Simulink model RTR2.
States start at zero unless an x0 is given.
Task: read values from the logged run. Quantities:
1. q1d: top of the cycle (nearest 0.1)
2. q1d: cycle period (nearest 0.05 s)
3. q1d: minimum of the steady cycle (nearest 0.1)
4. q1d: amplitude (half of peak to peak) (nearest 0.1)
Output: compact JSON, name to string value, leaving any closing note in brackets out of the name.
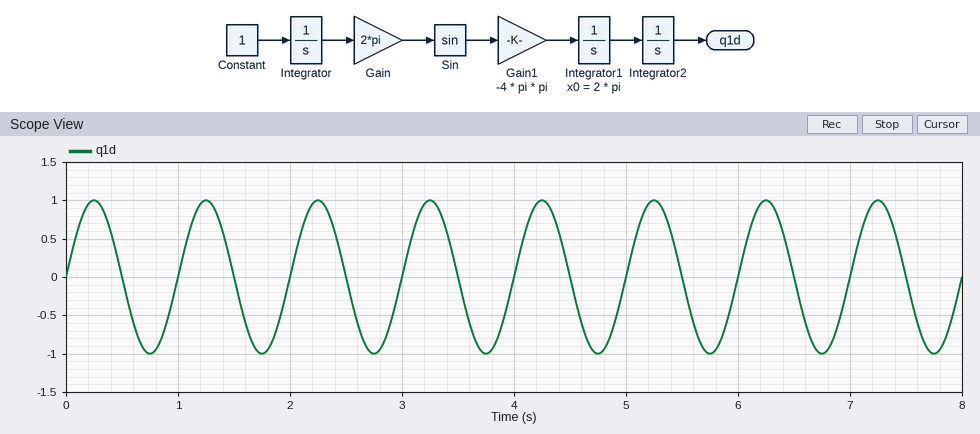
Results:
{"q1d: top of the cycle": "1.0", "q1d: cycle period": "1.00 s", "q1d: minimum of the steady cycle": "-1.0", "q1d: amplitude (half of peak to peak)": "1.0"}
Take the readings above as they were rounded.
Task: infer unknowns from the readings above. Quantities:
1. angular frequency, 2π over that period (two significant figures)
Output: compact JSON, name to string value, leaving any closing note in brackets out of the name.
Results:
{"angular frequency, 2π over that period": "6.3 rad/s"}
